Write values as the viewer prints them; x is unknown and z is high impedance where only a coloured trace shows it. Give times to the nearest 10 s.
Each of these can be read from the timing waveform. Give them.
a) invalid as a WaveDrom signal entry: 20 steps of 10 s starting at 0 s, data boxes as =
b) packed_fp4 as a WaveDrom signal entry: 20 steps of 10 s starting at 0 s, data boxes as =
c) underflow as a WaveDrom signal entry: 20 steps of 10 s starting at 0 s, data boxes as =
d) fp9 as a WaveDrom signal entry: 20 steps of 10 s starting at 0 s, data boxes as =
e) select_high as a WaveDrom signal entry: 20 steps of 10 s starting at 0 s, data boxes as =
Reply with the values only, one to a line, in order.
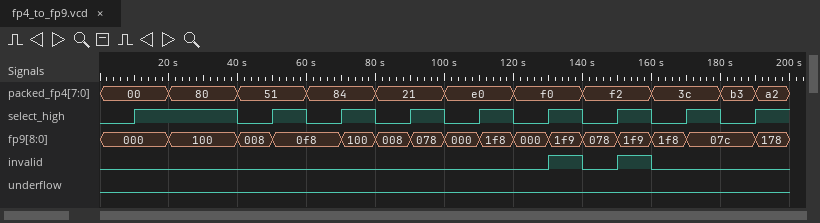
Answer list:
{name: 'invalid', wave: '0............1010...'}
{name: 'packed_fp4', wave: '=.=.=.=.=.=.=.=.=.==', data: '00 80 51 84 21 e0 f0 f2 3c b3 a2'}
{name: 'underflow', wave: '0...................'}
{name: 'fp9', wave: '=.=.==.===========.=', data: '000 100 008 0f8 100 008 078 000 1f8 000 1f9 078 1f9 1f8 07c 178'}
{name: 'select_high', wave: '01..0101010101010101'}
